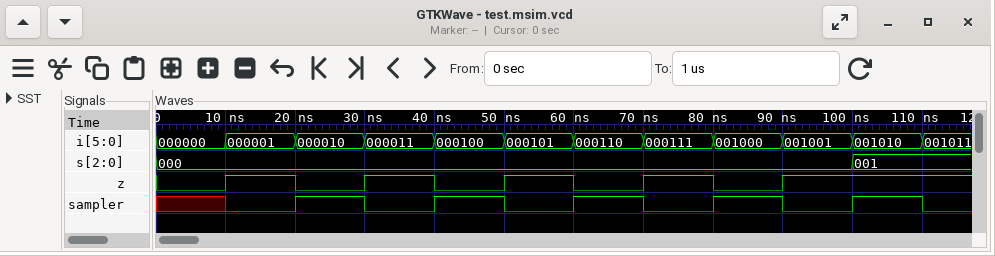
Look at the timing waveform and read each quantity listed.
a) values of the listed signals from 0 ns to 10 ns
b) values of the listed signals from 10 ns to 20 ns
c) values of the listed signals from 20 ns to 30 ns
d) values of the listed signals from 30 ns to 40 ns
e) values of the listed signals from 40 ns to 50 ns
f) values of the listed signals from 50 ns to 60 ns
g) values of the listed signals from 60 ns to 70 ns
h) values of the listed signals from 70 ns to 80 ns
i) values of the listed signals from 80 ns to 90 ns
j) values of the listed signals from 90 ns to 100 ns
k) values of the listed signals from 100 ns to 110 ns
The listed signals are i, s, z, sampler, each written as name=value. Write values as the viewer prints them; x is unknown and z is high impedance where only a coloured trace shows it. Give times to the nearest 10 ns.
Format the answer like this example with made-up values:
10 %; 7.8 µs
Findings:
i=000000, s=000, z=0, sampler=x; i=000001, s=000, z=1, sampler=0; i=000010, s=000, z=0, sampler=1; i=000011, s=000, z=1, sampler=0; i=000100, s=000, z=0, sampler=1; i=000101, s=000, z=1, sampler=0; i=000110, s=000, z=0, sampler=1; i=000111, s=000, z=1, sampler=0; i=001000, s=000, z=0, sampler=1; i=001001, s=000, z=1, sampler=0; i=001010, s=001, z=1, sampler=1
